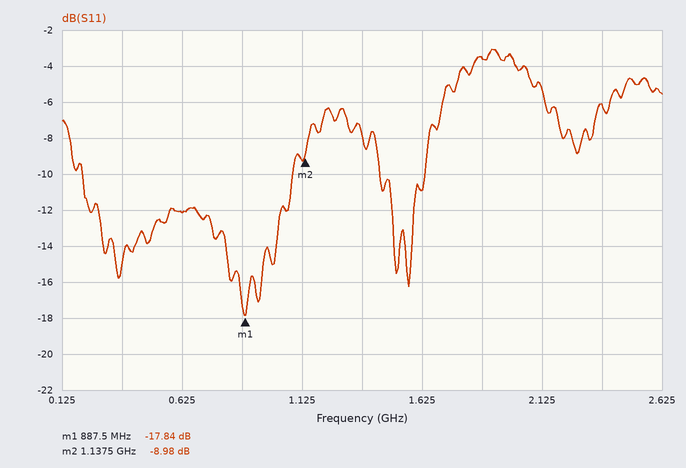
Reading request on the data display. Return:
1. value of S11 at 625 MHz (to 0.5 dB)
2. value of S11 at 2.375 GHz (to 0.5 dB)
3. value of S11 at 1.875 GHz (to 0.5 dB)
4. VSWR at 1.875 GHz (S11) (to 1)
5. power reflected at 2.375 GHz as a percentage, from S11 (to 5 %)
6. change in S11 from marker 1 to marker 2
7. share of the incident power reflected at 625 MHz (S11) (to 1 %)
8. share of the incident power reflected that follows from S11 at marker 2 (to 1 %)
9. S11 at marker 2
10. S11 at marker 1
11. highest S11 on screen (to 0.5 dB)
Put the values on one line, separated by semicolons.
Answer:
-12.0 dB; -6.0 dB; -3.5 dB; 5; 25 %; 8.86 dB; 6 %; 13 %; -8.98 dB; -17.84 dB; -3.0 dB
